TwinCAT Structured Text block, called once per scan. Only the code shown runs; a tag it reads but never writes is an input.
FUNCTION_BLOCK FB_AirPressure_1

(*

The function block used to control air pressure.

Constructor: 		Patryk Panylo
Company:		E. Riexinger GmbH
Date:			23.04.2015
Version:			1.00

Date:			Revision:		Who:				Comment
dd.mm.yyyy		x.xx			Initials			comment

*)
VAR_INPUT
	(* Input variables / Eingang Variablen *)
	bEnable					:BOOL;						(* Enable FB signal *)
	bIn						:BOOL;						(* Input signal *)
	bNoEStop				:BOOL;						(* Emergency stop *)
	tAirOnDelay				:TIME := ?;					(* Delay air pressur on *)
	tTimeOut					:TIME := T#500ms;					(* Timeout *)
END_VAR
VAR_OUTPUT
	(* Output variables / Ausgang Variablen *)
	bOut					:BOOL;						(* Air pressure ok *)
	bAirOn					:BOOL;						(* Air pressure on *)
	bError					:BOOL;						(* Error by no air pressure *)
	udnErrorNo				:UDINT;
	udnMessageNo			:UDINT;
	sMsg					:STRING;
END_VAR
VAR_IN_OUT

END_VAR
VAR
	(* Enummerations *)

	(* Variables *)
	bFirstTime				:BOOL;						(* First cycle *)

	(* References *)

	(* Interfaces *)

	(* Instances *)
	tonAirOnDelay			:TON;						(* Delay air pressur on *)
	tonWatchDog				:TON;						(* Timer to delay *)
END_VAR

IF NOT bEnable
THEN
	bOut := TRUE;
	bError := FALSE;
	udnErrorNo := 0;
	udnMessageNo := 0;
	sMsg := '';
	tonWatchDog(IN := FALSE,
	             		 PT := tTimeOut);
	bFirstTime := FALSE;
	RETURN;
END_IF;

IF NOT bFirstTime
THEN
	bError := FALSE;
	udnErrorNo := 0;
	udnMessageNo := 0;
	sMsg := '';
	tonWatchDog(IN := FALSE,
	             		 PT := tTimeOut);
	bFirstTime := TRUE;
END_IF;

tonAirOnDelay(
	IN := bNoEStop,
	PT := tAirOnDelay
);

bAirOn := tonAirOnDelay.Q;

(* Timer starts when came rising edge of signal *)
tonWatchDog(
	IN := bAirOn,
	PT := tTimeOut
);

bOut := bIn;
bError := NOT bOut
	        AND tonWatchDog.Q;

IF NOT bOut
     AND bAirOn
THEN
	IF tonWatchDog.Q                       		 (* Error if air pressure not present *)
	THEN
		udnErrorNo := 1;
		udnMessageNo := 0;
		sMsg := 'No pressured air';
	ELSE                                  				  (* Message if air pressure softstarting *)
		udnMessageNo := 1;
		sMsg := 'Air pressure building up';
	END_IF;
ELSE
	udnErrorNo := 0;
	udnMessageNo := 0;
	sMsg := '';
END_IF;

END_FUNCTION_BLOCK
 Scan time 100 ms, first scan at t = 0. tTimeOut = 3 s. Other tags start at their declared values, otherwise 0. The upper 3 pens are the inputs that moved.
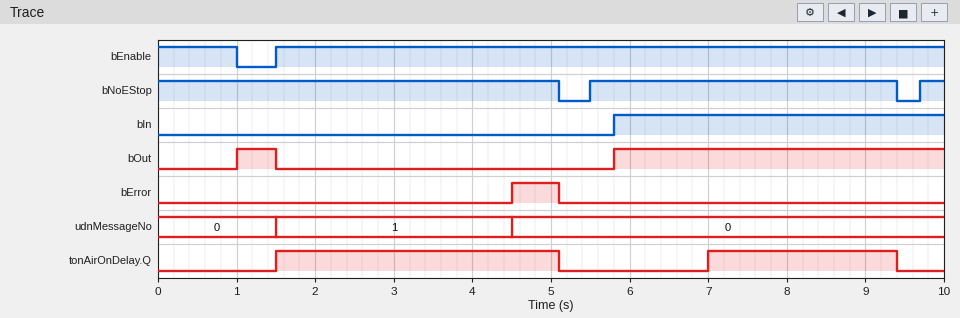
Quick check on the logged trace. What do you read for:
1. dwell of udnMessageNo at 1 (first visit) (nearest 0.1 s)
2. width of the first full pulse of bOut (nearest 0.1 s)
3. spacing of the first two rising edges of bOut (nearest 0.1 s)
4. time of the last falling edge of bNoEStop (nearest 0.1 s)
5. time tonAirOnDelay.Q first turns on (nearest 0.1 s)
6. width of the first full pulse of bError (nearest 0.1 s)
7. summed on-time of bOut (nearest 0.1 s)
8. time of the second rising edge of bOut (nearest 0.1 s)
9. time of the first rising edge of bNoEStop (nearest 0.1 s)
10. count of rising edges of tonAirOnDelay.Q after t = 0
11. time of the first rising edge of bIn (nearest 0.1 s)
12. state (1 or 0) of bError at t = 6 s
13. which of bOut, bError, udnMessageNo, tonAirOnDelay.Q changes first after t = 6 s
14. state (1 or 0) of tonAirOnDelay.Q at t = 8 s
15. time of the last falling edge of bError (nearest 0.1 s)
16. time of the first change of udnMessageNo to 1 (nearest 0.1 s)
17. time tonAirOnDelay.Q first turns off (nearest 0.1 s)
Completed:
3.0 s
0.5 s
4.8 s
9.4 s
1.5 s
0.6 s
4.7 s
5.8 s
5.5 s
2
5.8 s
0
tonAirOnDelay.Q
1
5.1 s
1.5 s
5.1 s
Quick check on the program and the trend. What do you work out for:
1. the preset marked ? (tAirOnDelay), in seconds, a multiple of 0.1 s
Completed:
1.5 s
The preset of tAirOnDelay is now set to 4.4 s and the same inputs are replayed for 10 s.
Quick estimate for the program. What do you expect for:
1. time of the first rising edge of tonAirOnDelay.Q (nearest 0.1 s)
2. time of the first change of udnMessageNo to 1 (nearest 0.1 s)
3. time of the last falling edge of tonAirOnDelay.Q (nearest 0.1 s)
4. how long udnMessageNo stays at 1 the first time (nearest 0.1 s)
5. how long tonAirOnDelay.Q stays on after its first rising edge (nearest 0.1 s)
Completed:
4.4 s
4.4 s
5.1 s
0.7 s
0.7 s
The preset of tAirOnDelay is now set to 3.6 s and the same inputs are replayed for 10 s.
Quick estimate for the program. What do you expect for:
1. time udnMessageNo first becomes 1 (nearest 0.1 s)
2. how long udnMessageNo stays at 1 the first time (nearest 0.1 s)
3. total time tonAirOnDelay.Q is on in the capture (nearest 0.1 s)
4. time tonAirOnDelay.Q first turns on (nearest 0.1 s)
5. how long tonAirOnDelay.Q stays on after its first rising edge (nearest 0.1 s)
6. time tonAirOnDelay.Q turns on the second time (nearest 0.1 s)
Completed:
3.6 s
1.5 s
1.8 s
3.6 s
1.5 s
9.1 s
